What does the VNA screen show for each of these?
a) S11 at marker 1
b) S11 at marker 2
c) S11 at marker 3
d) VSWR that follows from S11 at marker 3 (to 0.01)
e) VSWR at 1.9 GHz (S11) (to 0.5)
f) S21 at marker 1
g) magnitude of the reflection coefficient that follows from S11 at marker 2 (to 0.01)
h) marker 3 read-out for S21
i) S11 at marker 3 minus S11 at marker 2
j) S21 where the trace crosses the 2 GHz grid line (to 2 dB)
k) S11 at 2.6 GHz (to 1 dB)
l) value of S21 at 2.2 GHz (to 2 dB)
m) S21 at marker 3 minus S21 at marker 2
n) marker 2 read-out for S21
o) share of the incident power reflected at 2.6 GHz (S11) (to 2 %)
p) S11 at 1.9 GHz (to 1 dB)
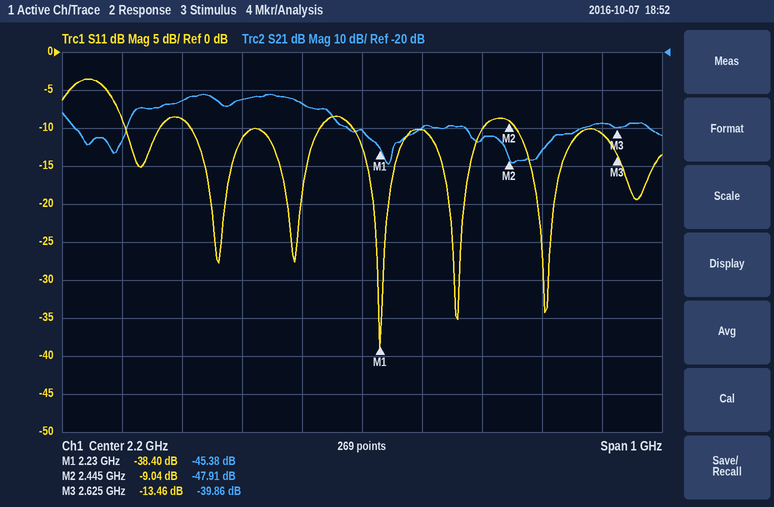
-38.40 dB
-9.04 dB
-13.46 dB
1.54
2.0
-45.38 dB
0.35
-39.86 dB
-4.42 dB
-32 dB
-11 dB
-40 dB
8.05 dB
-47.91 dB
8 %
-9 dB
